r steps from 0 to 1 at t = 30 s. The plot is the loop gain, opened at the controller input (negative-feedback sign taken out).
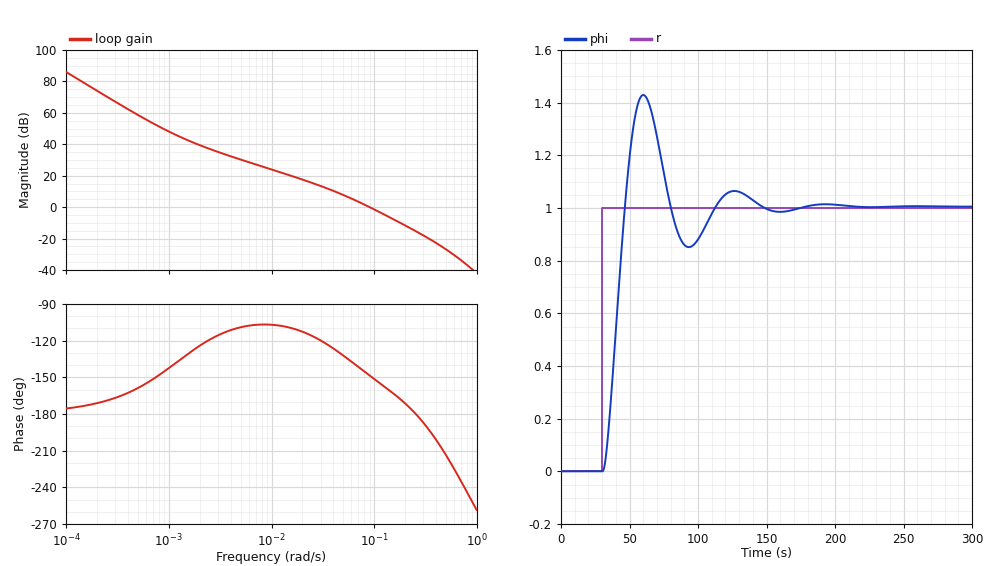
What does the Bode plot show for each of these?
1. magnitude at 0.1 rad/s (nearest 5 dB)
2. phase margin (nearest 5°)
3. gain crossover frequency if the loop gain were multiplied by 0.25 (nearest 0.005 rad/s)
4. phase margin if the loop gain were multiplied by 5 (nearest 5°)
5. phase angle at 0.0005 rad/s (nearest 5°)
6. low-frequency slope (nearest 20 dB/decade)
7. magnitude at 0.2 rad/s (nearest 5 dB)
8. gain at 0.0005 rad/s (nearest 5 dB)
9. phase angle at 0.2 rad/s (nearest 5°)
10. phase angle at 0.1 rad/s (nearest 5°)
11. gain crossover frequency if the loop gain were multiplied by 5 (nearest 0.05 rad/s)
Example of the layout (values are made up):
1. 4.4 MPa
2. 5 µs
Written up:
1. 0 dB
2. 30°
3. 0.035 rad/s
4. 5°
5. -160°
6. -40 dB/decade
7. -10 dB
8. 60 dB
9. -170°
10. -150°
11. 0.25 rad/s
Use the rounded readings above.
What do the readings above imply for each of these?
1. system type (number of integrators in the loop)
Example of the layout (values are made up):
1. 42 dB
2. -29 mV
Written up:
1. 2
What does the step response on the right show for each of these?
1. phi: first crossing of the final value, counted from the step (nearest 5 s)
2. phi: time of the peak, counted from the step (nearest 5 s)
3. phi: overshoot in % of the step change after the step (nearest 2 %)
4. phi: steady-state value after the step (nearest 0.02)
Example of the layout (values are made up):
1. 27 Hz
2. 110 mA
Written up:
1. 15 s
2. 30 s
3. 42 %
4. 1.00
